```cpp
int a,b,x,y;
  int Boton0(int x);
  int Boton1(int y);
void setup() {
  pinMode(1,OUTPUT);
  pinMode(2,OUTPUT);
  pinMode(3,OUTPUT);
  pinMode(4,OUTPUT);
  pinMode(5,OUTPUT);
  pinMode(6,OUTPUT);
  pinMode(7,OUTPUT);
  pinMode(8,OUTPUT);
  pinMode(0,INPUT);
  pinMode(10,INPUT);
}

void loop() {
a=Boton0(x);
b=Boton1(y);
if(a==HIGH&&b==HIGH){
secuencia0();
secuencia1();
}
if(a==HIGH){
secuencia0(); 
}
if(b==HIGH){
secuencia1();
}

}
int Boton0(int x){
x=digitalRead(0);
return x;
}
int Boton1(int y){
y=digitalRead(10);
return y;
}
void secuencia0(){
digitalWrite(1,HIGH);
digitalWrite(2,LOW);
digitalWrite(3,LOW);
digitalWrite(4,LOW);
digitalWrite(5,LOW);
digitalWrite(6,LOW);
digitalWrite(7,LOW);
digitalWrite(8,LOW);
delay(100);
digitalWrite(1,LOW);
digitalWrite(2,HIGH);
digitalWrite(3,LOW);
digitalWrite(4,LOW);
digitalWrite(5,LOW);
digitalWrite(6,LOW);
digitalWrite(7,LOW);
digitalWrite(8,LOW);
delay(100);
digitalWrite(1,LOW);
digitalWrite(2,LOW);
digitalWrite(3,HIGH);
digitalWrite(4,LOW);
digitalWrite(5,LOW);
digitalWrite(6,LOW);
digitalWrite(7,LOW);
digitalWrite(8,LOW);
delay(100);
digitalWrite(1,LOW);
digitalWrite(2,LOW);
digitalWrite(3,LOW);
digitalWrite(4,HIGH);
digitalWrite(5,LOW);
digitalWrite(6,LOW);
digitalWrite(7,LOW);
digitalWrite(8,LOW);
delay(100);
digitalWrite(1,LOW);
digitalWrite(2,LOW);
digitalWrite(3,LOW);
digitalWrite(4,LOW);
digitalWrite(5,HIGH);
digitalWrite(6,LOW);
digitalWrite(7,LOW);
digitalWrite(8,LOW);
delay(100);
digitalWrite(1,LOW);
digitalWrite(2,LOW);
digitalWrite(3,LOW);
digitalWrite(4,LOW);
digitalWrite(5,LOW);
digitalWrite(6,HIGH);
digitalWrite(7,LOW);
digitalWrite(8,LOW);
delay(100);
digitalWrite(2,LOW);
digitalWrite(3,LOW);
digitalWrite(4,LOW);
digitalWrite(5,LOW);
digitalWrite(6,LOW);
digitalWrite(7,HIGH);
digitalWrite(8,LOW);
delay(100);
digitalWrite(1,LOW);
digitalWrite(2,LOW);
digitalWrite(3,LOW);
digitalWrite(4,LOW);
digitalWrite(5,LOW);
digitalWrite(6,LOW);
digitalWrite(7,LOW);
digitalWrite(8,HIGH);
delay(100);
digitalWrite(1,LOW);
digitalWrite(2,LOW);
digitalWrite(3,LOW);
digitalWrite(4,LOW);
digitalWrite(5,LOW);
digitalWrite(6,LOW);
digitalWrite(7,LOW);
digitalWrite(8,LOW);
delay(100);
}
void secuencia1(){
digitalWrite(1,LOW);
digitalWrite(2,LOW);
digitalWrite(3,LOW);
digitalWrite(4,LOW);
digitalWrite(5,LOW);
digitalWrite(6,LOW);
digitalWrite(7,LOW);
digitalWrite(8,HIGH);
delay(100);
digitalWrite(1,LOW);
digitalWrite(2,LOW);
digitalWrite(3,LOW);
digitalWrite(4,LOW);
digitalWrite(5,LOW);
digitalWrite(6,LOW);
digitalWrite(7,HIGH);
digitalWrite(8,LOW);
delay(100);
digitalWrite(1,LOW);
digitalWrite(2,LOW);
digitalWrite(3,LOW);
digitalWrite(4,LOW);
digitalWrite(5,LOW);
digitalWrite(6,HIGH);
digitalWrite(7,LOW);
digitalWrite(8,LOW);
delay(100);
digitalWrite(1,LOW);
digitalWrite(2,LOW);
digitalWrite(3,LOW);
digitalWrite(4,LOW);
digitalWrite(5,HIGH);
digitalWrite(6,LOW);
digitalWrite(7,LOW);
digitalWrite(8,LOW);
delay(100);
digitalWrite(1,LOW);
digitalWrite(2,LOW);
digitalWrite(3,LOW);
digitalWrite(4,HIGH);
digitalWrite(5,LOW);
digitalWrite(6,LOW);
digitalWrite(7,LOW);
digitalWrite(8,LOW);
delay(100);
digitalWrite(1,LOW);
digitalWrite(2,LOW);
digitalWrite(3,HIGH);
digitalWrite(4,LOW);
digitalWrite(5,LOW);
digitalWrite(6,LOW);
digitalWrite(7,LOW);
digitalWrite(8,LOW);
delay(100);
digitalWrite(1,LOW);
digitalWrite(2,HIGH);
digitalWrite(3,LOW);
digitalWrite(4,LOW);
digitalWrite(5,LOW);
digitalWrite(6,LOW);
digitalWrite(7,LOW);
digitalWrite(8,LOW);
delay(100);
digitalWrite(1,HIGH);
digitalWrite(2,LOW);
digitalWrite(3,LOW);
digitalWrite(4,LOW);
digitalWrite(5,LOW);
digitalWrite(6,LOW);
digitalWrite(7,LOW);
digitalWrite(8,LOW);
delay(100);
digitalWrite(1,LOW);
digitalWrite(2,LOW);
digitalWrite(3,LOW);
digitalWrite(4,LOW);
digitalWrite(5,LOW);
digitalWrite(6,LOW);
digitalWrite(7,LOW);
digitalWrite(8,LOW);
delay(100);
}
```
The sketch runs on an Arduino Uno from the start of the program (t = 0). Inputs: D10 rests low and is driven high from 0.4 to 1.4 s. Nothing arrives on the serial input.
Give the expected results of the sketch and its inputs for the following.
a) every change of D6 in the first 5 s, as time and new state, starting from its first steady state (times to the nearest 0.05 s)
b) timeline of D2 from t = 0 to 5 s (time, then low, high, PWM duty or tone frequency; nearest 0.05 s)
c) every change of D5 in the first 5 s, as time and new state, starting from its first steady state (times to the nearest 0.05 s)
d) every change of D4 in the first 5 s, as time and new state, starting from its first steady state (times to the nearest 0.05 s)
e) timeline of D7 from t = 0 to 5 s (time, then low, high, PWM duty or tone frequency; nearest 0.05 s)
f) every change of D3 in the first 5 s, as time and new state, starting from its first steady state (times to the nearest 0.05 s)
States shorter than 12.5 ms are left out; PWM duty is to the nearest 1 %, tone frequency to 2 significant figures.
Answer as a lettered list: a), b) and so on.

a) 0 s low; 0.6 s high; 0.7 s low; 1.5 s high; 1.6 s low
b) 0 s low; 1 s high; 1.1 s low; 1.9 s high; 2 s low
c) 0 s low; 0.7 s high; 0.8 s low; 1.6 s high; 1.7 s low
d) 0 s low; 0.8 s high; 0.9 s low; 1.7 s high; 1.8 s low
e) 0 s low; 0.5 s high; 0.6 s low; 1.4 s high; 1.5 s low
f) 0 s low; 0.9 s high; 1 s low; 1.8 s high; 1.9 s low
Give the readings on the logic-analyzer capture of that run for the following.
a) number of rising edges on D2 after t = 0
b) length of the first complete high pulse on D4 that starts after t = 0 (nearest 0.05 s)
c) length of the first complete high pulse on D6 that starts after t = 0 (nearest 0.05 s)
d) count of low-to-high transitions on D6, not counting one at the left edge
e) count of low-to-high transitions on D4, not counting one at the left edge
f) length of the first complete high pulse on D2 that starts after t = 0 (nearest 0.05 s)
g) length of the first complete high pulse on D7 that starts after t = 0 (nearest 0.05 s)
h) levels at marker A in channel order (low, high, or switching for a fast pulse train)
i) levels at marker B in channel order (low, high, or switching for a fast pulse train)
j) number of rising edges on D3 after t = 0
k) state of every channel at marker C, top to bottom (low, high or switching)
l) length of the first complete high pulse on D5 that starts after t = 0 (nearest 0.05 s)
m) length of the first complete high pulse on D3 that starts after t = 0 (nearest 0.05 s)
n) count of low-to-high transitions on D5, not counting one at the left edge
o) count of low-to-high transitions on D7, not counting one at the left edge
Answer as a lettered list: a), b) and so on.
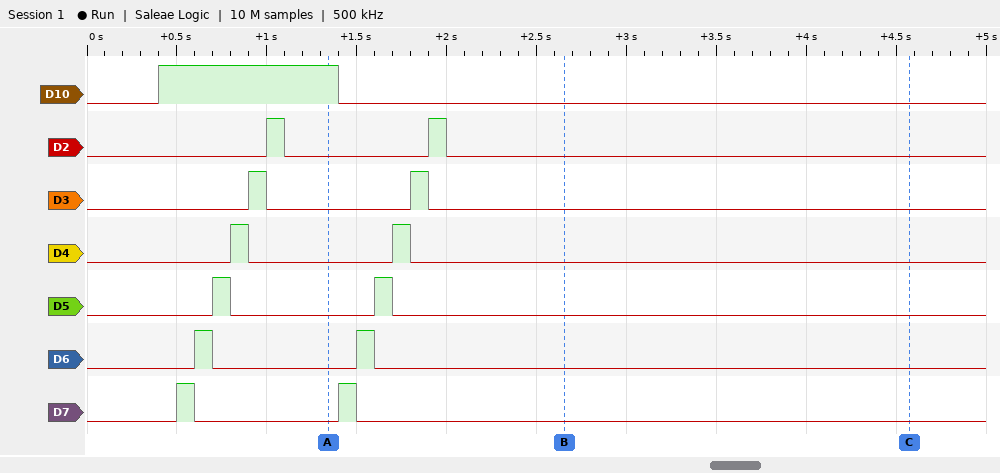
a) 2
b) 0.10 s
c) 0.10 s
d) 2
e) 2
f) 0.10 s
g) 0.10 s
h) D10 high, D2 low, D3 low, D4 low, D5 low, D6 low, D7 low
i) D10 low, D2 low, D3 low, D4 low, D5 low, D6 low, D7 low
j) 2
k) D10 low, D2 low, D3 low, D4 low, D5 low, D6 low, D7 low
l) 0.10 s
m) 0.10 s
n) 2
o) 2
